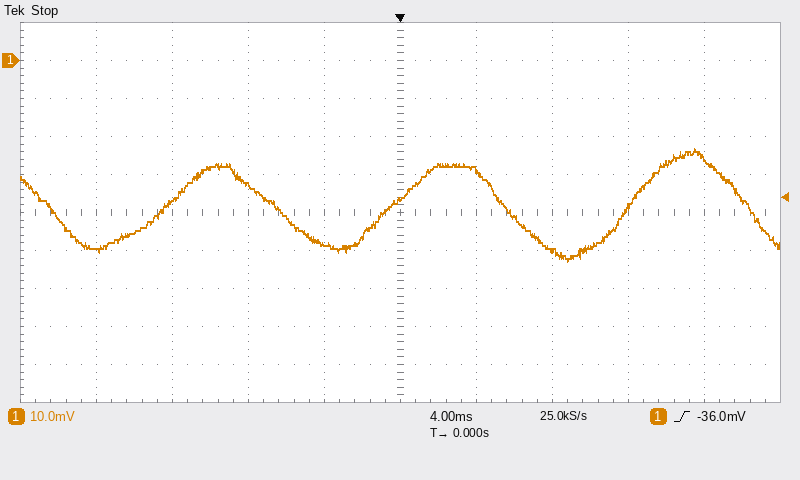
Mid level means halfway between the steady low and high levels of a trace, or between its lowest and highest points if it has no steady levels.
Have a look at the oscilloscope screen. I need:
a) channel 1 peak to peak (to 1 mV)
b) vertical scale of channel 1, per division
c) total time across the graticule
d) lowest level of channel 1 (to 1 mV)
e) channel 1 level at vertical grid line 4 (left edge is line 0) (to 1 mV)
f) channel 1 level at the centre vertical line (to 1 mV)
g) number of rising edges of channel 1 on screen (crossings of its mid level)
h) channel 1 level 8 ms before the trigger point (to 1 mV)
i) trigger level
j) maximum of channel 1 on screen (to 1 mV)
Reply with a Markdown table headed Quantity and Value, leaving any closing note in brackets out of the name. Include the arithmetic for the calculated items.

| Quantity | Value |
|---|---|
| channel 1 peak to peak | -23 mV − (-53 mV) = 30 mV |
| vertical scale of channel 1, per division | 10 mV |
| total time across the graticule | 40 ms |
| lowest level of channel 1 | -53 mV |
| channel 1 level at vertical grid line 4 (left edge is line 0) | -48 mV |
| channel 1 level at the centre vertical line | -37 mV |
| number of rising edges of channel 1 on screen | 3 |
| channel 1 level 8 ms before the trigger point | -33 mV |
| trigger level | -36.0 mV |
| maximum of channel 1 on screen | -23 mV |
